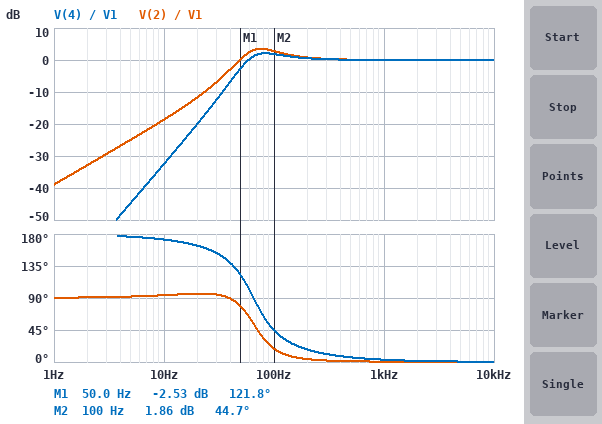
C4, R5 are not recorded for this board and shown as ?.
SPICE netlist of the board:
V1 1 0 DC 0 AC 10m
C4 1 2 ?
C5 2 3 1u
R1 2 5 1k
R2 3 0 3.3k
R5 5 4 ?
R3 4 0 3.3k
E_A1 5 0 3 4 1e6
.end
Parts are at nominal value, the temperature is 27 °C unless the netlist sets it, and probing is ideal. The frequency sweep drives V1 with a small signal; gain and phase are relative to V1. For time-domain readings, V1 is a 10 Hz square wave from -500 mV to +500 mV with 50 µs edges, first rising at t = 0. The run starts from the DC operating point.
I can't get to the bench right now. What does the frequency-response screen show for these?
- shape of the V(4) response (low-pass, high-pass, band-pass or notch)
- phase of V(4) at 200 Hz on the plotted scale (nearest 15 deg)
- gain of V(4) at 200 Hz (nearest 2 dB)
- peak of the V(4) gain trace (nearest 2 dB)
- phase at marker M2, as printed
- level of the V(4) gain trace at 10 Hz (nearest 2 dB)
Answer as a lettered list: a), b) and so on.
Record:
a) high-pass
b) 15 deg
c) 0 dB
d) 2 dB
e) 44.7 deg
f) -32 dB
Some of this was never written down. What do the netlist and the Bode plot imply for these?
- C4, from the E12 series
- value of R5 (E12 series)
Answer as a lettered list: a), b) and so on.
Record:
a) 1.8 µF
b) 680 Ω
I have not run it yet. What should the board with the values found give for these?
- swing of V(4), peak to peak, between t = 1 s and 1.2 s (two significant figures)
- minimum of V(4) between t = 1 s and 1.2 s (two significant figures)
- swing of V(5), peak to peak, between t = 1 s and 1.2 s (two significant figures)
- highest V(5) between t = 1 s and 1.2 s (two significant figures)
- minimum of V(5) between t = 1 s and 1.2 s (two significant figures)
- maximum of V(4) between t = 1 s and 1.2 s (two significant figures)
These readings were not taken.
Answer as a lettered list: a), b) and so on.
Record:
a) 2.0 V
b) -990 mV
c) 2.4 V
d) 1.2 V
e) -1.2 V
f) 990 mV
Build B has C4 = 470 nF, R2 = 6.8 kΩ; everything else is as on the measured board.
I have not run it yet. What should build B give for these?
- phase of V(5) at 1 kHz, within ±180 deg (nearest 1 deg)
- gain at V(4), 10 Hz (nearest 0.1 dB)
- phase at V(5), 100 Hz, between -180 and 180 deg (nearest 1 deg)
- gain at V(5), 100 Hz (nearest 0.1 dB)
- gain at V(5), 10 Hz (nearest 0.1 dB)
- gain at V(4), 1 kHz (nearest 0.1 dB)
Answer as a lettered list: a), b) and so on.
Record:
a) 0 deg
b) -37.9 dB
c) 9 deg
d) 15.2 dB
e) -36.2 dB
f) 0.1 dB
